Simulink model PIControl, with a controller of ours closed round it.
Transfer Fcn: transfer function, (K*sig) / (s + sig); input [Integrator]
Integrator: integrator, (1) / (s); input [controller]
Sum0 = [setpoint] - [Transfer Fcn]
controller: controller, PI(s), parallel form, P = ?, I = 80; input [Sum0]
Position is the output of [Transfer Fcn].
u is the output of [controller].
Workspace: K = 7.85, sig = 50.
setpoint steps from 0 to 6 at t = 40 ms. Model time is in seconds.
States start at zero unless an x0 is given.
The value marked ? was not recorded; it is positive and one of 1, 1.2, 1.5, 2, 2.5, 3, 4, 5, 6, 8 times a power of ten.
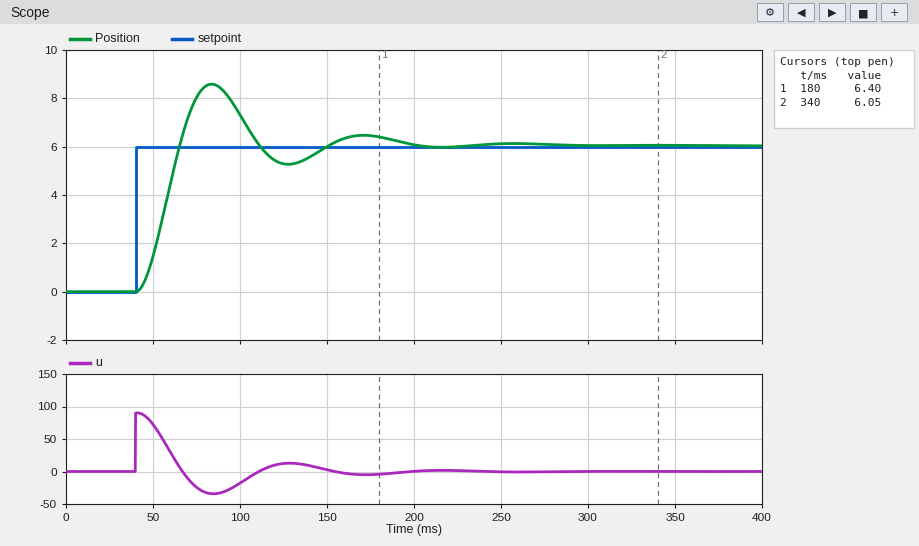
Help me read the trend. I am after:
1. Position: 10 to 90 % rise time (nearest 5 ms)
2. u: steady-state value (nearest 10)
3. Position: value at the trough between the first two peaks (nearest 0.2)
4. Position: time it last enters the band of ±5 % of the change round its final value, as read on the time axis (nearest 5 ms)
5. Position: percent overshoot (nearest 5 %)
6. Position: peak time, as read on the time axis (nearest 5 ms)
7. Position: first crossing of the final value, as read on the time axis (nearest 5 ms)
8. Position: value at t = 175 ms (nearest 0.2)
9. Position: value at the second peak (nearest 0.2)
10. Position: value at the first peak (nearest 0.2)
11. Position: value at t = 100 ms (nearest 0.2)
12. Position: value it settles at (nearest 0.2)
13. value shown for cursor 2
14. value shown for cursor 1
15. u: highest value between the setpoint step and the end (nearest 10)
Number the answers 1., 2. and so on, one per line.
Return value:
1. 15 ms
2. 0
3. 5.2
4. 185 ms
5. 45 %
6. 85 ms
7. 65 ms
8. 6.4
9. 6.4
10. 8.6
11. 7.4
12. 6.0
13. 6.05
14. 6.40
15. 90
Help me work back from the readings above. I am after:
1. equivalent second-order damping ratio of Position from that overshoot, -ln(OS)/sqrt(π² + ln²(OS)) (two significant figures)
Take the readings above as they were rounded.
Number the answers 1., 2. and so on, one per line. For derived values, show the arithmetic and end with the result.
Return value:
1. ln(0.45) = -0.799; 0.799 / sqrt(9.870 + 0.638) = 0.25
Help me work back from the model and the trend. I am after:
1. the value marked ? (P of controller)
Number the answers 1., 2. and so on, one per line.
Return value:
1. 15
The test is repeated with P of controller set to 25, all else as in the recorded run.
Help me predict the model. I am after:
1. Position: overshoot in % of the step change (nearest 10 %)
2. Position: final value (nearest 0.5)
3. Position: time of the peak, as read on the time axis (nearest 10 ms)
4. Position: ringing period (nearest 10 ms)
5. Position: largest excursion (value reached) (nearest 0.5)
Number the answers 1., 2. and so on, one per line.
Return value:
1. 50 %
2. 6.0
3. 70 ms
4. 70 ms
5. 9.0
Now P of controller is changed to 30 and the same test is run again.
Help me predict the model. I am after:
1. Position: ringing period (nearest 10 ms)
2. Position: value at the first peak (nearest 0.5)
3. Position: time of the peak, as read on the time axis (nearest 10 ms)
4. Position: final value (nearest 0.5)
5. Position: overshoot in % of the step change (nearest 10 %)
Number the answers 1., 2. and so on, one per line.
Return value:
1. 60 ms
2. 9.0
3. 70 ms
4. 6.0
5. 50 %
